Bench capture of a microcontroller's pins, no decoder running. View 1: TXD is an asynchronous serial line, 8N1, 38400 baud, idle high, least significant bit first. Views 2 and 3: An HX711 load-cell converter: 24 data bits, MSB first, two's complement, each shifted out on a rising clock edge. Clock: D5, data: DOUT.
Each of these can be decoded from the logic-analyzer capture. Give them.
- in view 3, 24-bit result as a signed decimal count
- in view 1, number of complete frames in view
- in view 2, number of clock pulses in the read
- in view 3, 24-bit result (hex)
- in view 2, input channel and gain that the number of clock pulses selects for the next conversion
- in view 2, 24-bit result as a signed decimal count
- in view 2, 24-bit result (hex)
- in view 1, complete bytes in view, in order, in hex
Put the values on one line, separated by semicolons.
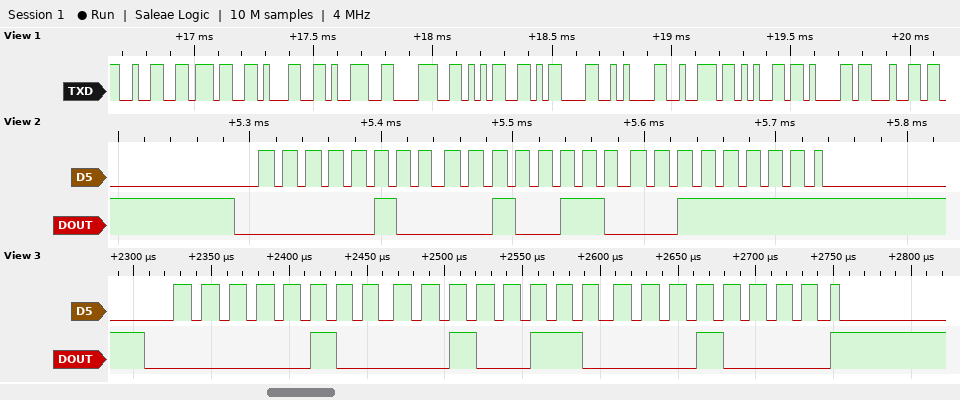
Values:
271888; 12; 25; 0x042610; channel A, gain 128; 271935; 0x04263F; 32 37 31 39 38 35 0D 0A 72 65 61 64
